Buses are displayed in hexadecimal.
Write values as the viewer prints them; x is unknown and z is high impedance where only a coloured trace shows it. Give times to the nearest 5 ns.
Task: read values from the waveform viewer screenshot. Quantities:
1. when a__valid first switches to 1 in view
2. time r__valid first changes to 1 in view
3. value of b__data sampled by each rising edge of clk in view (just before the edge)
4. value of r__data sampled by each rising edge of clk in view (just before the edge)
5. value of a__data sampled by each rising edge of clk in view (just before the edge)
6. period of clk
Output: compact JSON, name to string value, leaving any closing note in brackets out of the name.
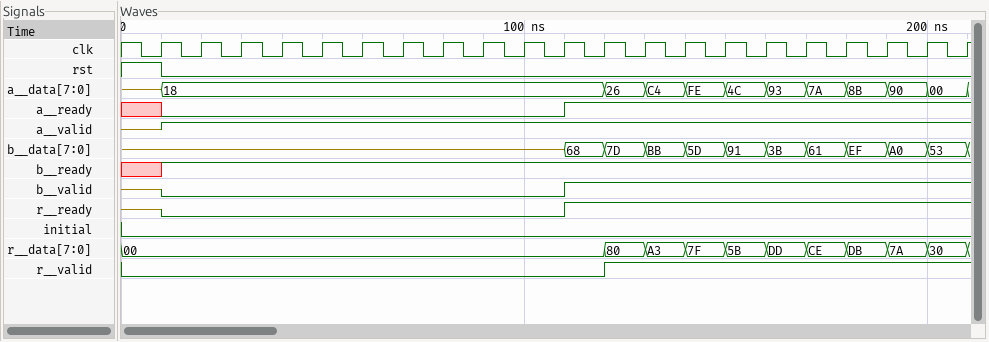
{"when a__valid first switches to 1 in view": "10 ns", "time r__valid first changes to 1 in view": "120 ns", "value of b__data sampled by each rising edge of clk in view": "z, z, z, z, z, z, z, z, z, z, z, 68, 7D, BB, 5D, 91, 3B, 61, EF, A0, 53", "value of r__data sampled by each rising edge of clk in view": "00, 00, 00, 00, 00, 00, 00, 00, 00, 00, 00, 00, 80, A3, 7F, 5B, DD, CE, DB, 7A, 30", "value of a__data sampled by each rising edge of clk in view": "z, 18, 18, 18, 18, 18, 18, 18, 18, 18, 18, 18, 26, C4, FE, 4C, 93, 7A, 8B, 90, 00", "period of clk": "10 ns"}
